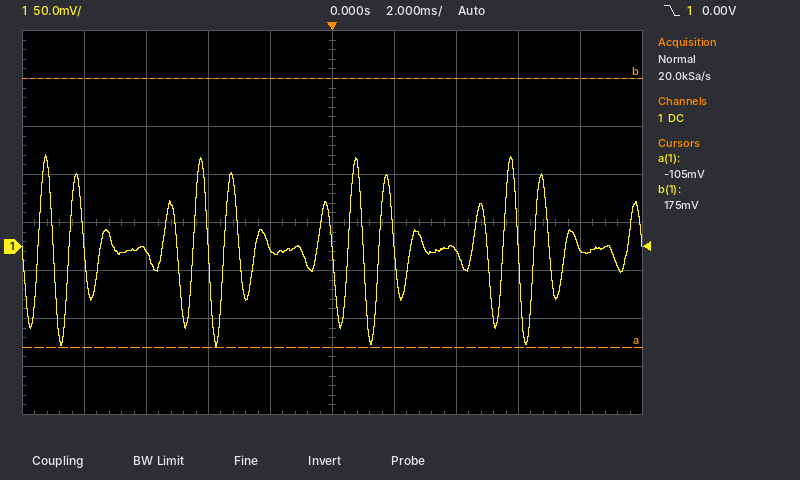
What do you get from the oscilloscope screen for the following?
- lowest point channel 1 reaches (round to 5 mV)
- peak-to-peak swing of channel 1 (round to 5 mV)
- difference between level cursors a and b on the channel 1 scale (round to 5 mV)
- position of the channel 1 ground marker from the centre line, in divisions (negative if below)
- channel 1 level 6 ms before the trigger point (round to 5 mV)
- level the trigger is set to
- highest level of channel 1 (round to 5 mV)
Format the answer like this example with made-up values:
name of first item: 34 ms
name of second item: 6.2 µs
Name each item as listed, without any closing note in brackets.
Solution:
lowest point channel 1 reaches: -105 mV
peak-to-peak swing of channel 1: 200 mV
difference between level cursors a and b on the channel 1 scale: 280 mV
position of the channel 1 ground marker from the centre line, in divisions: -0.5 div
channel 1 level 6 ms before the trigger point: -5 mV
level the trigger is set to: 0.00 V
highest level of channel 1: 95 mV
